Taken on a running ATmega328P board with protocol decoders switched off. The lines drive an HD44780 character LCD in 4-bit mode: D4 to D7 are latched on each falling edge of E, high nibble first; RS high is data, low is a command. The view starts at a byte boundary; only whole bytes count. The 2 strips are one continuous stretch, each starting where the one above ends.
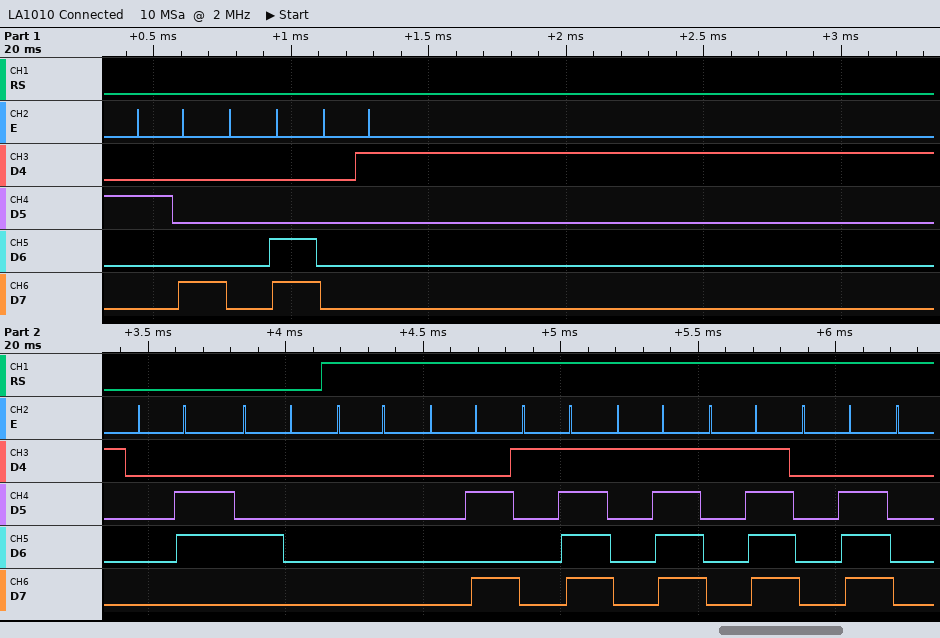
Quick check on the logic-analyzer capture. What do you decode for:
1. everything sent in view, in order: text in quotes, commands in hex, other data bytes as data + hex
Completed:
0x28 0x0C 0x01 0x06 0x40 data 00 0A 1F 1F 1F 0E
